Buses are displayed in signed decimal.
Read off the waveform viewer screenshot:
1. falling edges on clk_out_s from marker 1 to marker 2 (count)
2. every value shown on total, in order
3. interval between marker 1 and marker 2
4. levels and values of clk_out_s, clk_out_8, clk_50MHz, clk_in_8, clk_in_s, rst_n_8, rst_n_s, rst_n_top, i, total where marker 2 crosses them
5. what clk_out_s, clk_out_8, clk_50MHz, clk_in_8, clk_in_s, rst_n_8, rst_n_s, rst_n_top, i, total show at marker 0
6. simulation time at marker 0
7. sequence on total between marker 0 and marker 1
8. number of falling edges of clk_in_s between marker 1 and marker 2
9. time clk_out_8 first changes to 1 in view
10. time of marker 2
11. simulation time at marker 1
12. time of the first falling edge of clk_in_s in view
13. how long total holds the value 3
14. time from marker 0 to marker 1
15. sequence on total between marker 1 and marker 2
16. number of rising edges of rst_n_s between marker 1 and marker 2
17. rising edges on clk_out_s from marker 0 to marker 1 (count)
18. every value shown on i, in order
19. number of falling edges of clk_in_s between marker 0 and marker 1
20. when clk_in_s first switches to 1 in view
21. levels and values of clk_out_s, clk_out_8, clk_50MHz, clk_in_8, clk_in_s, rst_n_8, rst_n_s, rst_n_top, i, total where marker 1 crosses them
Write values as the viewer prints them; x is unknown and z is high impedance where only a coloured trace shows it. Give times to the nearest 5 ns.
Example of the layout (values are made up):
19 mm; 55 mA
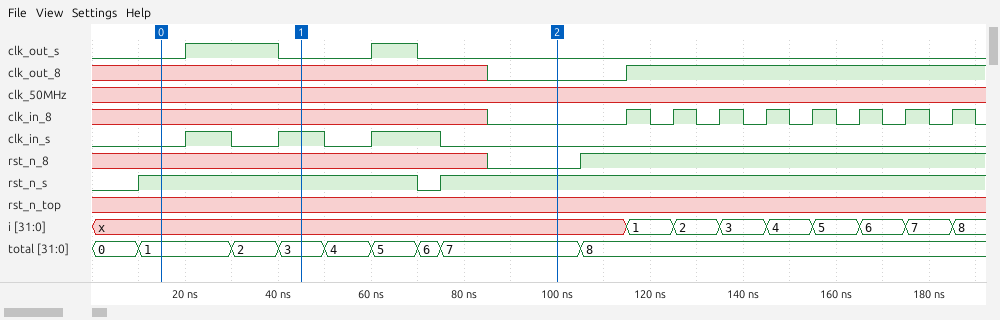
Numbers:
1; 0, 1, 2, 3, 4, 5, 6, 7, 8; 55 ns; clk_out_s=0, clk_out_8=0, clk_50MHz=x, clk_in_8=0, clk_in_s=0, rst_n_8=0, rst_n_s=1, rst_n_top=x, i=x, total=7; clk_out_s=0, clk_out_8=x, clk_50MHz=x, clk_in_8=x, clk_in_s=0, rst_n_8=x, rst_n_s=1, rst_n_top=x, i=x, total=1; 15 ns; 1, 2, 3; 2; 115 ns; 100 ns; 45 ns; 30 ns; 10 ns; 30 ns; 3, 4, 5, 6, 7; 1; 1; x, 1, 2, 3, 4, 5, 6, 7, 8; 1; 20 ns; clk_out_s=0, clk_out_8=x, clk_50MHz=x, clk_in_8=x, clk_in_s=1, rst_n_8=x, rst_n_s=1, rst_n_top=x, i=x, total=3
